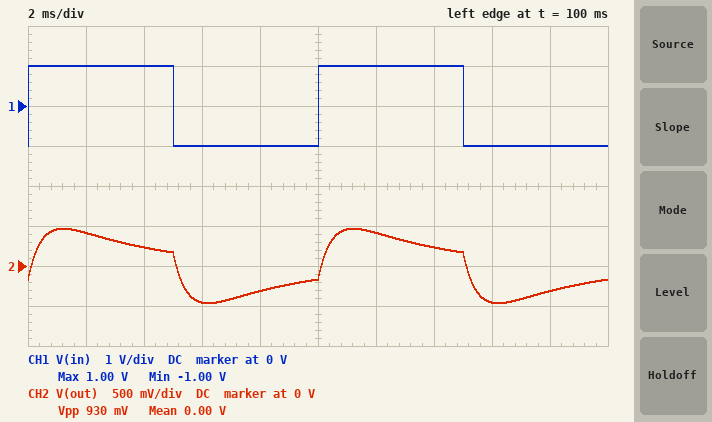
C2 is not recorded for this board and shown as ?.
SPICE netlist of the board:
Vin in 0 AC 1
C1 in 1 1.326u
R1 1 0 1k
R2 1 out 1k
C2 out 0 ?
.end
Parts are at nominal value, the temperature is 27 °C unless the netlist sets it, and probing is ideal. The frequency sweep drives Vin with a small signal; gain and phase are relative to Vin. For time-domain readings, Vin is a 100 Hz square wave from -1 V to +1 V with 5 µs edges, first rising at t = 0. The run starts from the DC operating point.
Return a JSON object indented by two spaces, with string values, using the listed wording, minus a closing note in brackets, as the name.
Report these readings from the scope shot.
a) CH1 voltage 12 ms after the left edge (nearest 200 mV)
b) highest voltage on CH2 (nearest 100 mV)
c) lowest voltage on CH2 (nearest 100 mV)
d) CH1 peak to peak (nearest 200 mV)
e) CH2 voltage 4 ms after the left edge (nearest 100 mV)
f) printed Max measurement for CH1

{
  "CH1 voltage 12 ms after the left edge": "1.0 V",
  "highest voltage on CH2": "500 mV",
  "lowest voltage on CH2": "-500 mV",
  "CH1 peak to peak": "2.0 V",
  "CH2 voltage 4 ms after the left edge": "200 mV",
  "printed Max measurement for CH1": "1.00 V"
}
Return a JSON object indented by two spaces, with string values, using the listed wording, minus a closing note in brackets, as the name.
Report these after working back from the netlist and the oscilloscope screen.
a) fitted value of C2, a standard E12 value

{
  "fitted value of C2, a standard E12 value": "1.2 µF"
}
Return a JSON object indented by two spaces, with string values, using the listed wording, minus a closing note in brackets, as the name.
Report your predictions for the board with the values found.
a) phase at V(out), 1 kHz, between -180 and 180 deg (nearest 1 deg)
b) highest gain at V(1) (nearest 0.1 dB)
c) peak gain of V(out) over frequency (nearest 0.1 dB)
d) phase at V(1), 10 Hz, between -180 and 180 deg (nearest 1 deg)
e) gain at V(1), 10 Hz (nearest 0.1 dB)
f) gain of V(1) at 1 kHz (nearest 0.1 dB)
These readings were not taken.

{
  "phase at V(out), 1 kHz, between -180 and 180 deg": "-69 deg",
  "highest gain at V(1)": "0 dB",
  "peak gain of V(out) over frequency": "-9.0 dB",
  "phase at V(1), 10 Hz, between -180 and 180 deg": "81 deg",
  "gain at V(1), 10 Hz": "-21.7 dB",
  "gain of V(1) at 1 kHz": "-0.4 dB"
}
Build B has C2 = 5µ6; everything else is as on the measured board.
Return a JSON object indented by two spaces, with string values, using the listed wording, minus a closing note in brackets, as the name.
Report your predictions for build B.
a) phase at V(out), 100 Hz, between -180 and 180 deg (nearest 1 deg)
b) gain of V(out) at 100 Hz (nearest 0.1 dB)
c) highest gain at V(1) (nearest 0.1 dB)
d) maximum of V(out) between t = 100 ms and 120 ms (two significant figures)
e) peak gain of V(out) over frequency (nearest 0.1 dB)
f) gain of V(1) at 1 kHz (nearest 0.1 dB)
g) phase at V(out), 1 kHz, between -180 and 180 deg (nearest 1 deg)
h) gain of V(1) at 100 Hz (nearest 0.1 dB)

{
  "phase at V(out), 100 Hz, between -180 and 180 deg": "-14 deg",
  "gain of V(out) at 100 Hz": "-19.8 dB",
  "highest gain at V(1)": "0 dB",
  "maximum of V(out) between t = 100 ms and 120 ms": "110 mV",
  "peak gain of V(out) over frequency": "-19.5 dB",
  "gain of V(1) at 1 kHz": "-0.3 dB",
  "phase at V(out), 1 kHz, between -180 and 180 deg": "-75 deg",
  "gain of V(1) at 100 Hz": "-8.5 dB"
}
